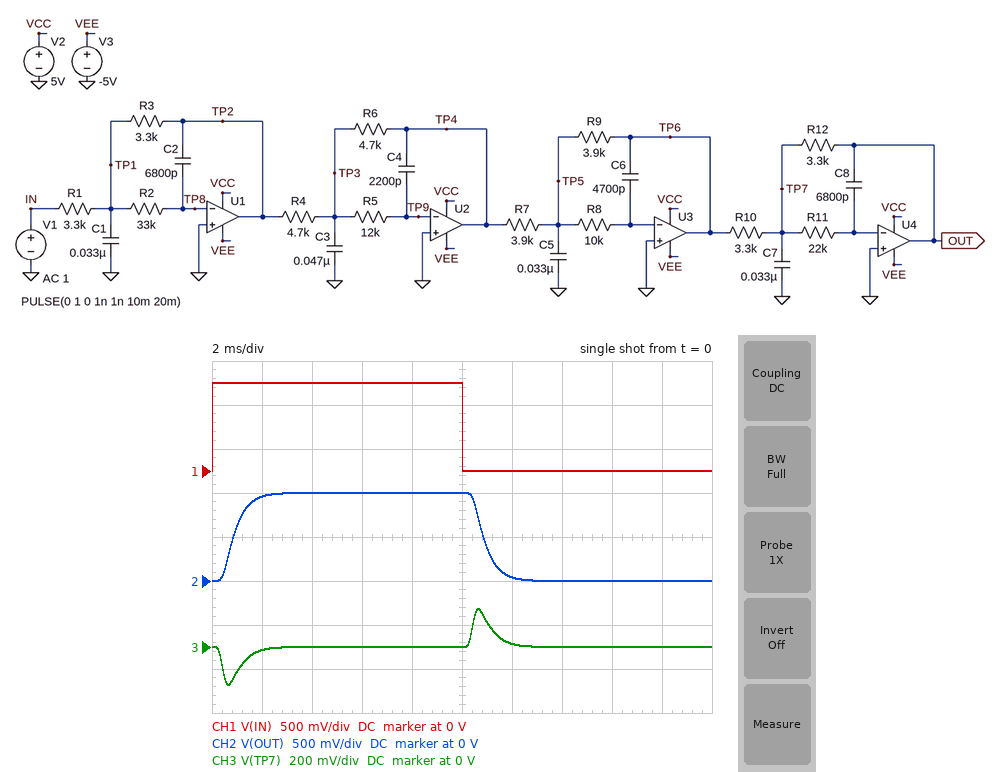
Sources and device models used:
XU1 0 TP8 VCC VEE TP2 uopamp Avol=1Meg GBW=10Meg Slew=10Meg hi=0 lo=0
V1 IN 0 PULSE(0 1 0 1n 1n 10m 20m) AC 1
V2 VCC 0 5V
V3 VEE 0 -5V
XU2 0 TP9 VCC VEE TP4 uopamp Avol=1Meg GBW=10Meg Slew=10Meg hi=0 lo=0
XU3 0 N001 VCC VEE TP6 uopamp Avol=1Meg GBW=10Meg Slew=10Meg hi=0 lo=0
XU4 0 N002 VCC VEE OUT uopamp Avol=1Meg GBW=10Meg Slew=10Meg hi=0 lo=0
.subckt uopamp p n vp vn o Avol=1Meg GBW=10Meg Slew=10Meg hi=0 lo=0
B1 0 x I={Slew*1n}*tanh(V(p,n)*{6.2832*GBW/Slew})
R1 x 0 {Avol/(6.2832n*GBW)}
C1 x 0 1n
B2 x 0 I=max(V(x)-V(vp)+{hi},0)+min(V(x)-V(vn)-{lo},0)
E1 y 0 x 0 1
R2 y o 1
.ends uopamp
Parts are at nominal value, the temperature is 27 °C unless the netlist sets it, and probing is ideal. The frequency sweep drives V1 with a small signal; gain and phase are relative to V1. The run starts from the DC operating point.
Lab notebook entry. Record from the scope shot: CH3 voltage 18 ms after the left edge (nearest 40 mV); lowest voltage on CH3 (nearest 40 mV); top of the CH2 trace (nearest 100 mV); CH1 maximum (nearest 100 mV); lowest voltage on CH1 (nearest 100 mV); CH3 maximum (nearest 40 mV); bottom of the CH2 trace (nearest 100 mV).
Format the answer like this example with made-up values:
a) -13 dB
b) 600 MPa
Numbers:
a) 0 V
b) -160 mV
c) 1.0 V
d) 1.0 V
e) 0 V
f) 160 mV
g) 0 V
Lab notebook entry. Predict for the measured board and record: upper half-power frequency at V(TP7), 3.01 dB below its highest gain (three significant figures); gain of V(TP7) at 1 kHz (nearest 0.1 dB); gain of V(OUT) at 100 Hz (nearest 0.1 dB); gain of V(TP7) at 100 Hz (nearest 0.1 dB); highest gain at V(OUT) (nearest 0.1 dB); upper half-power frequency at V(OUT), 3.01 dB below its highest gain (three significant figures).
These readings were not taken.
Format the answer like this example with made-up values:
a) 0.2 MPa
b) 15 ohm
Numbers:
a) 1.12 kHz
b) -15.3 dB
c) -0.4 dB
d) -20.9 dB
e) 0 dB
f) 302 Hz
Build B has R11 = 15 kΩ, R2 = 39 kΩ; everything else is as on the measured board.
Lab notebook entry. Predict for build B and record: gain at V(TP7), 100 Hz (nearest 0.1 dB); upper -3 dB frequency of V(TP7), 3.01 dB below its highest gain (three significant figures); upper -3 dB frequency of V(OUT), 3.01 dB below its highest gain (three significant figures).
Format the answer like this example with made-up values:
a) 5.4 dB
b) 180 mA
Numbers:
a) -24.3 dB
b) 1.31 kHz
c) 295 Hz
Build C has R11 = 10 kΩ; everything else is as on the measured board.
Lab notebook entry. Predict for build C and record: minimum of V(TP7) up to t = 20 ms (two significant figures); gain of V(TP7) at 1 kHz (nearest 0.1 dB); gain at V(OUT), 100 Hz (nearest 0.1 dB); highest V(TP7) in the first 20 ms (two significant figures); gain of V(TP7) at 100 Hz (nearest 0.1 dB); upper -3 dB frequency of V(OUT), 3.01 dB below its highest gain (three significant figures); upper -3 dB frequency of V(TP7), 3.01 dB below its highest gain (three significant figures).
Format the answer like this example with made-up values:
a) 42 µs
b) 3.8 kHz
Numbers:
a) -110 mV
b) -17.6 dB
c) -0.3 dB
d) 110 mV
e) -27.7 dB
f) 372 Hz
g) 1.59 kHz
